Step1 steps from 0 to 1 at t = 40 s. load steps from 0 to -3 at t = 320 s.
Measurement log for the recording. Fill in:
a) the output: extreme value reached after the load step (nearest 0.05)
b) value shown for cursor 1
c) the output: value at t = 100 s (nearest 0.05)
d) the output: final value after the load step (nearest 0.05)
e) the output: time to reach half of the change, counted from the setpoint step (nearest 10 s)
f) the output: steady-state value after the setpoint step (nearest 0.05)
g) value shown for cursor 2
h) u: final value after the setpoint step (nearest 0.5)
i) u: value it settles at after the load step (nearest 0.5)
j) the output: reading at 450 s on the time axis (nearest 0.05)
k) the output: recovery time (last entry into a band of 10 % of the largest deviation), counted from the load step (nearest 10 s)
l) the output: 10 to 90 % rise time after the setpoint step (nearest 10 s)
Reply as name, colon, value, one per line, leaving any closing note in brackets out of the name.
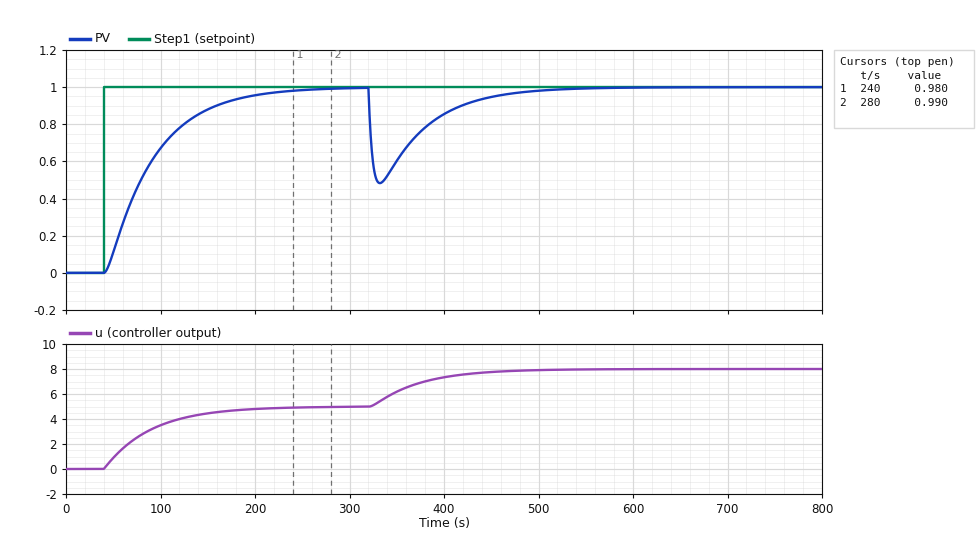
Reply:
the output: extreme value reached after the load step: 0.50
value shown for cursor 1: 0.980
the output: value at t = 100 s: 0.65
the output: final value after the load step: 1.00
the output: time to reach half of the change, counted from the setpoint step: 40 s
the output: steady-state value after the setpoint step: 1.00
value shown for cursor 2: 0.990
u: final value after the setpoint step: 5.0
u: value it settles at after the load step: 8.0
the output: reading at 450 s on the time axis: 0.95
the output: recovery time (last entry into a band of 10 % of the largest deviation), counted from the load step: 130 s
the output: 10 to 90 % rise time after the setpoint step: 110 s
